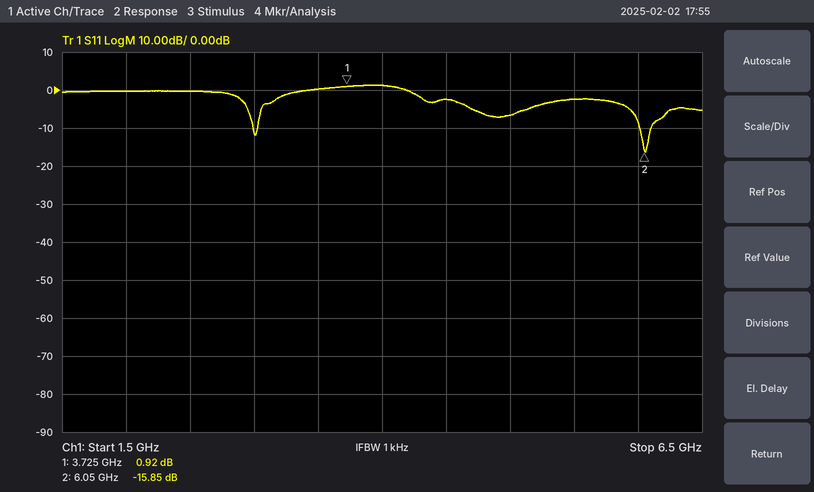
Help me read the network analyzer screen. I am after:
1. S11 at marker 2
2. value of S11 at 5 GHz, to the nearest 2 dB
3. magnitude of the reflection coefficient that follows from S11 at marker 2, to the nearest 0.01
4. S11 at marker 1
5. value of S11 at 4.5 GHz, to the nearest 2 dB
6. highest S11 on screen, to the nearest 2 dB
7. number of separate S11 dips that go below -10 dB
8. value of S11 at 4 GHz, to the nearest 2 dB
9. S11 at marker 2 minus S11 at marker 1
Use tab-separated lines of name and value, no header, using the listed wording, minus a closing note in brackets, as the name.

S11 at marker 2	-15.85 dB
value of S11 at 5 GHz, to the nearest 2 dB	-6 dB
magnitude of the reflection coefficient that follows from S11 at marker 2, to the nearest 0.01	0.16
S11 at marker 1	0.92 dB
value of S11 at 4.5 GHz, to the nearest 2 dB	-2 dB
highest S11 on screen, to the nearest 2 dB	2 dB
number of separate S11 dips that go below -10 dB	2
value of S11 at 4 GHz, to the nearest 2 dB	2 dB
S11 at marker 2 minus S11 at marker 1	-16.77 dB
